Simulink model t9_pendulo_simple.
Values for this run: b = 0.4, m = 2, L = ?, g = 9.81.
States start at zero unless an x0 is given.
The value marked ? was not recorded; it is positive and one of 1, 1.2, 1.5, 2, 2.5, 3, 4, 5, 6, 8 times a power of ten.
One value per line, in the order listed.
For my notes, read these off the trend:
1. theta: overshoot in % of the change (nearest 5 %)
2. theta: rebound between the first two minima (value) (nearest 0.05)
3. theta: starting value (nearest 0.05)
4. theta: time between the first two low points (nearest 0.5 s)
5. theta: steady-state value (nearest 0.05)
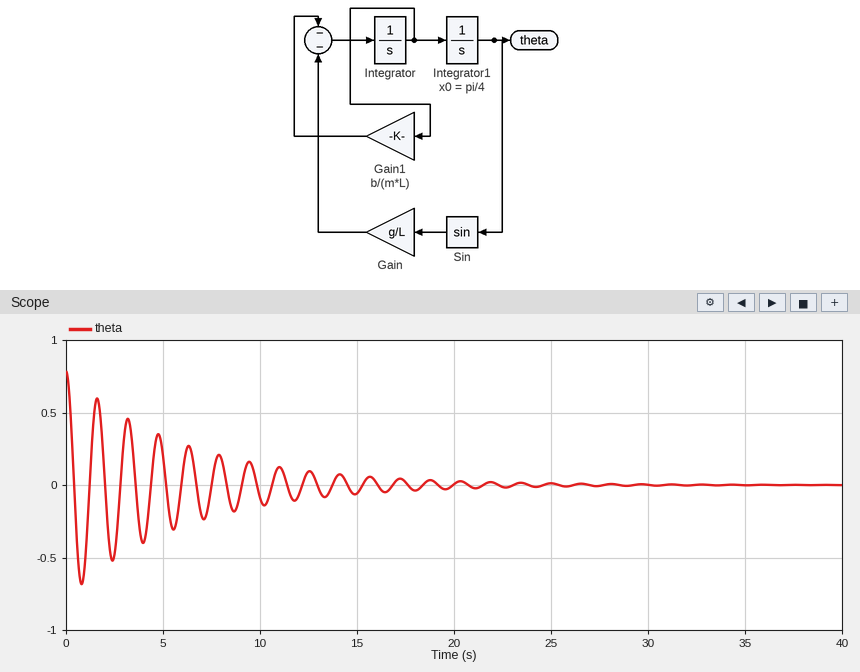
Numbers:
85 %
0.60
0.80
1.5 s
0.00
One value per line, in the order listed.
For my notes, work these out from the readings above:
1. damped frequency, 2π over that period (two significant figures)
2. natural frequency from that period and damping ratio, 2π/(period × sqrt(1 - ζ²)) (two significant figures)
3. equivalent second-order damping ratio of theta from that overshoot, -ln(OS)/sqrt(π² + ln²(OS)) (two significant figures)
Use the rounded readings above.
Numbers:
4.2 rad/s
4.2 rad/s
0.052
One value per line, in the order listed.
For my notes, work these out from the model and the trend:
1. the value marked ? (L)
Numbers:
0.6
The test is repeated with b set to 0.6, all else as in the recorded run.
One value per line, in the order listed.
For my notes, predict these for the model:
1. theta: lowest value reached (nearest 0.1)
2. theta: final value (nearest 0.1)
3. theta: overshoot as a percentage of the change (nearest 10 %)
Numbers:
-0.6
0.0
80 %
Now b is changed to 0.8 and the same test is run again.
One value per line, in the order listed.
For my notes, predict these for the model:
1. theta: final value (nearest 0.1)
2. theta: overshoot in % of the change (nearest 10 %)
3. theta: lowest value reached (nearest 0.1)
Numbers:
0.0
80 %
-0.6
